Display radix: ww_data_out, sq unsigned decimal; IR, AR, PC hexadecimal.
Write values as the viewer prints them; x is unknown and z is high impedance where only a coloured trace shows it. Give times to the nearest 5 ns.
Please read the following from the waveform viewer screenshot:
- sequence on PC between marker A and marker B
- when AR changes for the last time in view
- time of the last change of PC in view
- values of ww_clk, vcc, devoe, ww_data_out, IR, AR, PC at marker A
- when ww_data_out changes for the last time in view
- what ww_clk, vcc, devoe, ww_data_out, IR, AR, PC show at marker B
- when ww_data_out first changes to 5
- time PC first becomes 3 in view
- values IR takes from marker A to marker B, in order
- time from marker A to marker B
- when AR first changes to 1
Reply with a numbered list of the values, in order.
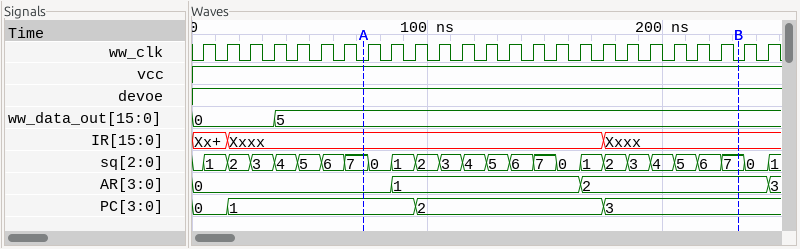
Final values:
1. 1, 2, 3
2. 245 ns
3. 175 ns
4. ww_clk=0, vcc=1, devoe=1, ww_data_out=5, IR=Xxxx, AR=0, PC=1
5. 35 ns
6. ww_clk=0, vcc=1, devoe=1, ww_data_out=5, IR=Xxxx, AR=2, PC=3
7. 35 ns
8. 175 ns
9. Xxxx, Xxxx
10. 160 ns
11. 85 ns
